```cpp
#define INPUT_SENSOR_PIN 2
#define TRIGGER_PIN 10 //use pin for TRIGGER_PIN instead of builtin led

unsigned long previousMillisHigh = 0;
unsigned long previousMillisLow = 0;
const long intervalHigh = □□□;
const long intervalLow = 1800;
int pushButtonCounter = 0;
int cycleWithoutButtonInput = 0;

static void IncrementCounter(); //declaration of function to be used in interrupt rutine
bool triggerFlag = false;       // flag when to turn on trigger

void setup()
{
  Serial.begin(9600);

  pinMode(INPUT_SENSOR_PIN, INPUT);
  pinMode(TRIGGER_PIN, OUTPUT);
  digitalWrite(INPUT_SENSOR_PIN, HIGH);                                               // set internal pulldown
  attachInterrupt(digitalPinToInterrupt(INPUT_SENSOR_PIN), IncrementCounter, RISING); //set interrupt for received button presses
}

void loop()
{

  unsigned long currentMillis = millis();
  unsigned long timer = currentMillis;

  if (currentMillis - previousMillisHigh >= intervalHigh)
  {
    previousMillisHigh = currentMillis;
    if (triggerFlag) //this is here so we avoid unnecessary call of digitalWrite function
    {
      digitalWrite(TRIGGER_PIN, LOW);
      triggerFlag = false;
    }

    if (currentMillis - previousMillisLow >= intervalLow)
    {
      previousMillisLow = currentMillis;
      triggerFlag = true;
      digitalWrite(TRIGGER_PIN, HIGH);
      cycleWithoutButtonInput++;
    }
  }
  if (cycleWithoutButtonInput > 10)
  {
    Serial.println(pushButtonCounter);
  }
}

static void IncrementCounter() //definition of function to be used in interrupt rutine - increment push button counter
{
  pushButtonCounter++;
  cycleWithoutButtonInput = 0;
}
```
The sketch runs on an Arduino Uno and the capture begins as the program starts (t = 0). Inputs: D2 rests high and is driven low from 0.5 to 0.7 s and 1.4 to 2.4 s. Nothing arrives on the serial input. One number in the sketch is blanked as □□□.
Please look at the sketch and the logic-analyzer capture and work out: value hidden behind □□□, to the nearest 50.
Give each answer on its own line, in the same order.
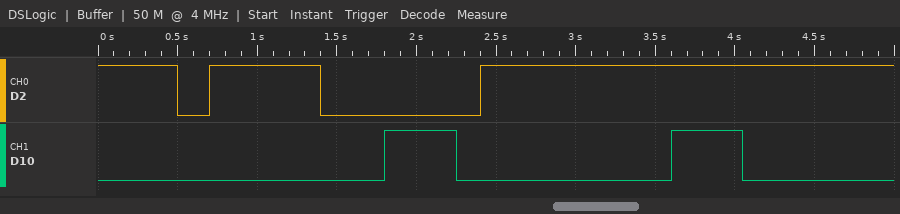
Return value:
450
